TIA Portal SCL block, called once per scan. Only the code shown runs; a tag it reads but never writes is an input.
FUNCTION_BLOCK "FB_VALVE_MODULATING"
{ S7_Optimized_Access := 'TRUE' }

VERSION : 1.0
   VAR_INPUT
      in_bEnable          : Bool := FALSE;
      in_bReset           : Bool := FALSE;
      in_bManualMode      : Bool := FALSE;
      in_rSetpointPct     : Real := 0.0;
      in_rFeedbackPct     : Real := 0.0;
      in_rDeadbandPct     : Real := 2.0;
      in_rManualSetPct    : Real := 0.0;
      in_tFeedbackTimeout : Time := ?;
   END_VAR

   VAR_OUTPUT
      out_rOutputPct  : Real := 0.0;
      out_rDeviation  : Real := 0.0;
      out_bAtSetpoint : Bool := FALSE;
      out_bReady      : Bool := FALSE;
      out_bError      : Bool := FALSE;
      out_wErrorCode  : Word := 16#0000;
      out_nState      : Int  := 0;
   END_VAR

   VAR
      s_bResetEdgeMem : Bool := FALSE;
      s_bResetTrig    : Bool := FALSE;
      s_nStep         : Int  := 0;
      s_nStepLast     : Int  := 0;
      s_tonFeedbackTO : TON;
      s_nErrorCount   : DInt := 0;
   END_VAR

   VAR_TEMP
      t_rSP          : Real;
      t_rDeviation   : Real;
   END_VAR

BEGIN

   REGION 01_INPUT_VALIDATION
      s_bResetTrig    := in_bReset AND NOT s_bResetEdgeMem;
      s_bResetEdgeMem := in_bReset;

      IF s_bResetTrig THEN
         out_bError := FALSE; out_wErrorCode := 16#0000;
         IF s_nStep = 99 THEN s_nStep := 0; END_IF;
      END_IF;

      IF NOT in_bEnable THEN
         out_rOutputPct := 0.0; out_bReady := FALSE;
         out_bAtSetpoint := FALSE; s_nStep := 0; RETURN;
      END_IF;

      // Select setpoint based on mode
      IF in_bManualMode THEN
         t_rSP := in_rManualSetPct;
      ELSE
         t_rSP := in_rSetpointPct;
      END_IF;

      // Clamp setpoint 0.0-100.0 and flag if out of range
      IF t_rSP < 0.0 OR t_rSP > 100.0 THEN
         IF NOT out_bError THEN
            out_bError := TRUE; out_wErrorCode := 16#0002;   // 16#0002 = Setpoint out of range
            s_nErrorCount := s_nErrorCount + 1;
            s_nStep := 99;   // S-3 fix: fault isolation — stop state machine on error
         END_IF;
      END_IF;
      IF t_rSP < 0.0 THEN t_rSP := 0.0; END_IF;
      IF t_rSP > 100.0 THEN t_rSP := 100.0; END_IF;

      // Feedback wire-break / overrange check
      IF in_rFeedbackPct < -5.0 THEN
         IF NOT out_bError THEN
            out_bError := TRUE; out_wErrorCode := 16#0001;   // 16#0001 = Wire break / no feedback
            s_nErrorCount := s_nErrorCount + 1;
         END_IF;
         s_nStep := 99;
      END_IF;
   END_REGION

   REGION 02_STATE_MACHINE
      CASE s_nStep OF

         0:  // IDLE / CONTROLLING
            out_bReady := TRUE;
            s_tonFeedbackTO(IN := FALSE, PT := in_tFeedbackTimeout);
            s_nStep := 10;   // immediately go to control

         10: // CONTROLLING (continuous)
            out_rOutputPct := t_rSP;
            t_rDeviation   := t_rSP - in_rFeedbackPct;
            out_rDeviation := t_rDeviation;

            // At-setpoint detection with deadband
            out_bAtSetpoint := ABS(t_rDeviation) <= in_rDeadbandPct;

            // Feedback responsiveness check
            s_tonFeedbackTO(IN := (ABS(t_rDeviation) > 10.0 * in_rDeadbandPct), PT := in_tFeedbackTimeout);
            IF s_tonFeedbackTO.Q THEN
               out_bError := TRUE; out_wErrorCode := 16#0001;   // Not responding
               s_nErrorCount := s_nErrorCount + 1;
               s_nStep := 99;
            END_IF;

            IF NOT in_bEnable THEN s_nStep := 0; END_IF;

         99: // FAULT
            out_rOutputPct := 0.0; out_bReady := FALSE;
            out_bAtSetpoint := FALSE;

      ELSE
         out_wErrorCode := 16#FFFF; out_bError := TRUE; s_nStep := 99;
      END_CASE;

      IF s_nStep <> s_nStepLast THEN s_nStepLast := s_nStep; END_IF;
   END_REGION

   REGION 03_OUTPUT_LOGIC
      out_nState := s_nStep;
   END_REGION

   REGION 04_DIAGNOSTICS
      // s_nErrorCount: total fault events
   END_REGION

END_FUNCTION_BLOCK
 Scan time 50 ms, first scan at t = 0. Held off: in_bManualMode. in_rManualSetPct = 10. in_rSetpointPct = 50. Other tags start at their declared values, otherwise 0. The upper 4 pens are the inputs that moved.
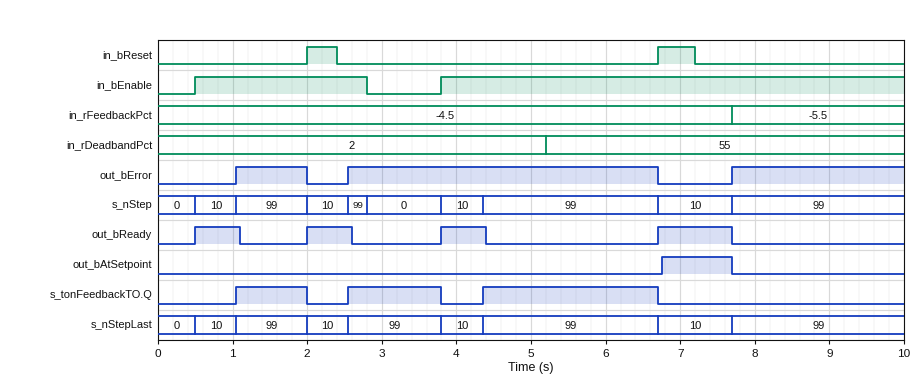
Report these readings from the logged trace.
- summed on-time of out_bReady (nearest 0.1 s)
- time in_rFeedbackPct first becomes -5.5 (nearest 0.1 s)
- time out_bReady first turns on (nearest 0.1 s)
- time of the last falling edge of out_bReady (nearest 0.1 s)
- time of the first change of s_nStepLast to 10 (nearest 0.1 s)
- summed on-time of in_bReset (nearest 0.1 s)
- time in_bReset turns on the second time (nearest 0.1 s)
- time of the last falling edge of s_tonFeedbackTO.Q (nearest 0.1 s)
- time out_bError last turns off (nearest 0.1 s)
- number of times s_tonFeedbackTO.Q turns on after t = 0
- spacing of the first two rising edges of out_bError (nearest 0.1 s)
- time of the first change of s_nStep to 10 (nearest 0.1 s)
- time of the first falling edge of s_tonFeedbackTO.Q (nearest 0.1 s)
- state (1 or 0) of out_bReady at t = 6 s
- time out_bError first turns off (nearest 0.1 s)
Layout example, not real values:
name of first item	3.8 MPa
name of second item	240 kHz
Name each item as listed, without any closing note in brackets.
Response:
summed on-time of out_bReady	2.8 s
time in_rFeedbackPct first becomes -5.5	7.7 s
time out_bReady first turns on	0.5 s
time of the last falling edge of out_bReady	7.7 s
time of the first change of s_nStepLast to 10	0.5 s
summed on-time of in_bReset	0.9 s
time in_bReset turns on the second time	6.7 s
time of the last falling edge of s_tonFeedbackTO.Q	6.7 s
time out_bError last turns off	6.7 s
number of times s_tonFeedbackTO.Q turns on after t = 0	3
spacing of the first two rising edges of out_bError	1.5 s
time of the first change of s_nStep to 10	0.5 s
time of the first falling edge of s_tonFeedbackTO.Q	2.0 s
state (1 or 0) of out_bReady at t = 6 s	0
time out_bError first turns off	2.0 s
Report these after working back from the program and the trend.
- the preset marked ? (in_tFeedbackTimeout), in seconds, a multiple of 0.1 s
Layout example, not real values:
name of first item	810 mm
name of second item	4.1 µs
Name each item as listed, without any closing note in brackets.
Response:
the preset marked ? (in_tFeedbackTimeout), in seconds, a multiple of 0.1 s	0.5 s
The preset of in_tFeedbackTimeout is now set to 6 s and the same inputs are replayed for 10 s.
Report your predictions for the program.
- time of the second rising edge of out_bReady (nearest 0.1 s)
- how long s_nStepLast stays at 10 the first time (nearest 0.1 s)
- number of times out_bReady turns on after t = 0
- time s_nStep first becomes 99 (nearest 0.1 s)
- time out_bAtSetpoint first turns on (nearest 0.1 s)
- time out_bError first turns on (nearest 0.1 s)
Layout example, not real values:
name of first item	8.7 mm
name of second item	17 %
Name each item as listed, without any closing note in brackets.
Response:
time of the second rising edge of out_bReady	3.8 s
how long s_nStepLast stays at 10 the first time	7.2 s
number of times out_bReady turns on after t = 0	2
time s_nStep first becomes 99	7.7 s
time out_bAtSetpoint first turns on	5.2 s
time out_bError first turns on	7.7 s
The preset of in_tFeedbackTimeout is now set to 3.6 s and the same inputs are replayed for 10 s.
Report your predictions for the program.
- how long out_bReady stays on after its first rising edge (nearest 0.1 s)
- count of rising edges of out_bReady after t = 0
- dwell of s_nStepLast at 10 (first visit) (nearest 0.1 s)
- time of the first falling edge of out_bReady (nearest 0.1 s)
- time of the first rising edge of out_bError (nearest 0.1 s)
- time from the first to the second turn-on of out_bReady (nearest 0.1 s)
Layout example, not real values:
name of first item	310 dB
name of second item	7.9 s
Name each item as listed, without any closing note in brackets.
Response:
how long out_bReady stays on after its first rising edge	2.3 s
count of rising edges of out_bReady after t = 0	2
dwell of s_nStepLast at 10 (first visit)	7.2 s
time of the first falling edge of out_bReady	2.8 s
time of the first rising edge of out_bError	7.7 s
time from the first to the second turn-on of out_bReady	3.3 s
